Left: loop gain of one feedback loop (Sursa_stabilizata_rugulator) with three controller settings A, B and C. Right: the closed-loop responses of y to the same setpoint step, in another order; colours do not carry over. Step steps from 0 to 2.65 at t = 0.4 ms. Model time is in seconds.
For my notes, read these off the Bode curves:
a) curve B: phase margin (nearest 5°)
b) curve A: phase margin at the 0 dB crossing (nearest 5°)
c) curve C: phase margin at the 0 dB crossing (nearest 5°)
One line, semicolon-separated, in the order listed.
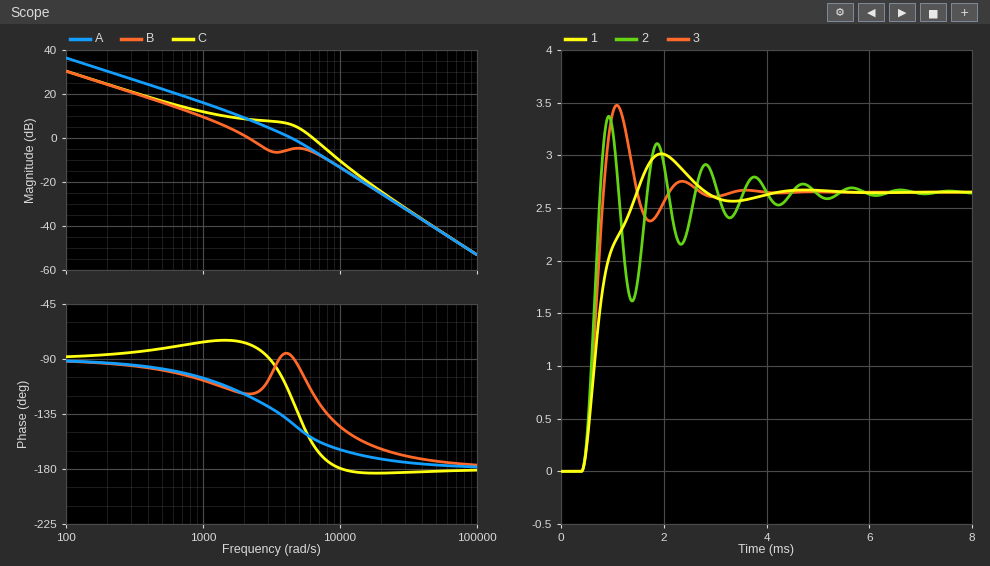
60°; 40°; 20°
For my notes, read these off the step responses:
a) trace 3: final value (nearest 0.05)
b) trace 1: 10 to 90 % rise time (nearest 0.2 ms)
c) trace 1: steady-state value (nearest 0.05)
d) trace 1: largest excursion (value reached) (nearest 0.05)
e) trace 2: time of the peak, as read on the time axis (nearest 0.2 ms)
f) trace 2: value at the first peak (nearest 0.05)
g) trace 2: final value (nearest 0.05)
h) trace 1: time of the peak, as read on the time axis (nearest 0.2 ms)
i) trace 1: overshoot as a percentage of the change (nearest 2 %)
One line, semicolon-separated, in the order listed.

2.65; 0.8 ms; 2.65; 3.00; 1.0 ms; 3.35; 2.65; 2.0 ms; 14 %
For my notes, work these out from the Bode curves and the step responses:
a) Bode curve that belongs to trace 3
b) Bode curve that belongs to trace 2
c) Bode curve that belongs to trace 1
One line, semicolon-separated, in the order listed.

A; C; B
